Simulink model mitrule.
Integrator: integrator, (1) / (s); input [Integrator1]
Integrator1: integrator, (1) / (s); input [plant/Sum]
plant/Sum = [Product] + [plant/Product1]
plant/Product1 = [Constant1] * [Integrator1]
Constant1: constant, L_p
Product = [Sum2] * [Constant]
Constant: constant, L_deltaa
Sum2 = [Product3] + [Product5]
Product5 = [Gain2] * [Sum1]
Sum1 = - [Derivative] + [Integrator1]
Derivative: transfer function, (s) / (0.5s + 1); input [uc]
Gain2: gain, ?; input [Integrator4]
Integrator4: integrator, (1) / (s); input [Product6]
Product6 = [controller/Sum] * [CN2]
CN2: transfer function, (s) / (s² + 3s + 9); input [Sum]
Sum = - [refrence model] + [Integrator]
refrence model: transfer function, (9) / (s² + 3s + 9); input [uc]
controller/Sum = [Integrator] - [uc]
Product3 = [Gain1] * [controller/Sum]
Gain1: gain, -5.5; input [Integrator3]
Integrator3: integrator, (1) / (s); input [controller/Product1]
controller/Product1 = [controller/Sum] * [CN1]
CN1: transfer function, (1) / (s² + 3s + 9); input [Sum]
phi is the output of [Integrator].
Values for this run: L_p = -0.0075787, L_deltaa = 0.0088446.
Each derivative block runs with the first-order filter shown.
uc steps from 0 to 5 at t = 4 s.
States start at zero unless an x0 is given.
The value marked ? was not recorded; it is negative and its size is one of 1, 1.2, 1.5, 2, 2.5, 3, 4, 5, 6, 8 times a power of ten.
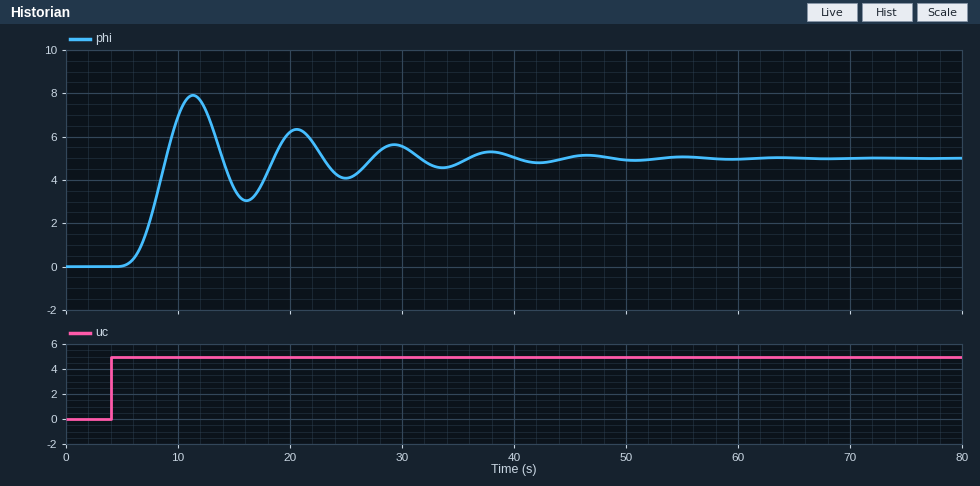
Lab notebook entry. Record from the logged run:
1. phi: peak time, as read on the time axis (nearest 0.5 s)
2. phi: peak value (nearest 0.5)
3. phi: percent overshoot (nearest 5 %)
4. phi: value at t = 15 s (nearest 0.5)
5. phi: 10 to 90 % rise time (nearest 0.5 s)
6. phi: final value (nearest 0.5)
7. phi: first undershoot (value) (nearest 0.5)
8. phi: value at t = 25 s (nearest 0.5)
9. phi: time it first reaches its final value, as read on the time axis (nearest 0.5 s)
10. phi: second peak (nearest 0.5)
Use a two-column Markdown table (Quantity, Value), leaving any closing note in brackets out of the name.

| Quantity | Value |
|---|---|
| phi: peak time, as read on the time axis | 11.5 s |
| phi: peak value | 8.0 |
| phi: percent overshoot | 60 % |
| phi: value at t = 15 s | 3.5 |
| phi: 10 to 90 % rise time | 2.5 s |
| phi: final value | 5.0 |
| phi: first undershoot (value) | 3.0 |
| phi: value at t = 25 s | 4.0 |
| phi: time it first reaches its final value, as read on the time axis | 9.0 s |
| phi: second peak | 6.5 |
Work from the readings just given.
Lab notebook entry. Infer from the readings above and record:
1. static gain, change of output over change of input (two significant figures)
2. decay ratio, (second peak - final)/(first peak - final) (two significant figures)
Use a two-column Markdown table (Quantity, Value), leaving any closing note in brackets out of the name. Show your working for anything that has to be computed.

| Quantity | Value |
|---|---|
| static gain, change of output over change of input | (5 - 0) / (5 - 0) = 1.0 |
| decay ratio, (second peak - final)/(first peak - final) | (6.5 - 5) / (8 - 5) = 0.50 |
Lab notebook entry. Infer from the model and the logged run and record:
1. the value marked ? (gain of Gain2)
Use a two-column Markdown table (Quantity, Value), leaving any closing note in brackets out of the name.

| Quantity | Value |
|---|---|
| the value marked ? | -8 |
